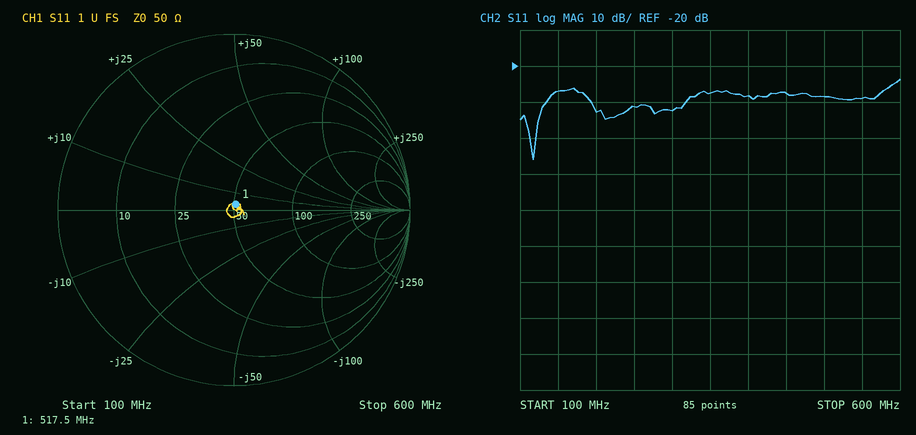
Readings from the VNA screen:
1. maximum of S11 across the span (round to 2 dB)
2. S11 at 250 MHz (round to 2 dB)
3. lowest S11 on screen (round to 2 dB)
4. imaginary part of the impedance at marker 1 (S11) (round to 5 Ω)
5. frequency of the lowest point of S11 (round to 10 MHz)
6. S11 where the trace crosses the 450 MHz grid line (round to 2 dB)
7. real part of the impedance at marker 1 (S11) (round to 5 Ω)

-24 dB
-32 dB
-46 dB
+5 Ω
120 MHz
-28 dB
50 Ω
